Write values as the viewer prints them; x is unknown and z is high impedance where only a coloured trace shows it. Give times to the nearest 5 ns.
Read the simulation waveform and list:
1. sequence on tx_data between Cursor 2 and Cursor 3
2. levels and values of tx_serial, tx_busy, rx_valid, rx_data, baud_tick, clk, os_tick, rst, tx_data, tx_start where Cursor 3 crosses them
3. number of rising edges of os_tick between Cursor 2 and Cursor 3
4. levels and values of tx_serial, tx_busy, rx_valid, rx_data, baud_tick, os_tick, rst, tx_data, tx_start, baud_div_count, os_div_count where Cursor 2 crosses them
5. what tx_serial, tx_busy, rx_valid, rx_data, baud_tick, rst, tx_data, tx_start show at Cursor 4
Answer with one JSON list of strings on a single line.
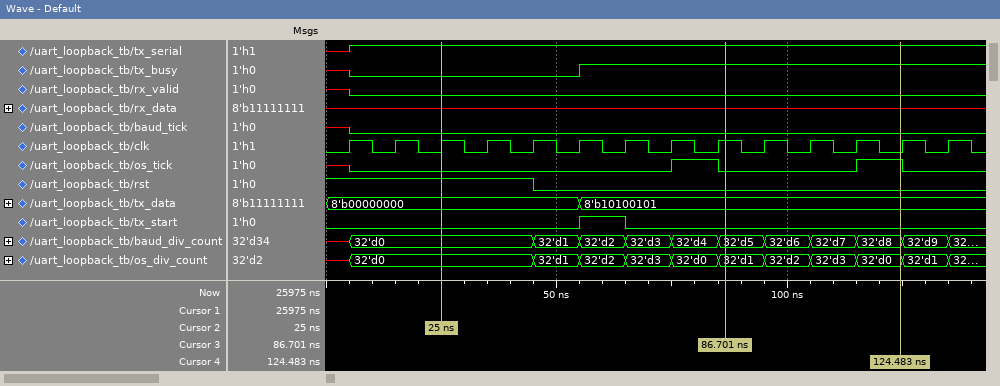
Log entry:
["8'b00000000, 8'b10100101", "tx_serial=1, tx_busy=1, rx_valid=0, rx_data=x, baud_tick=0, clk=1, os_tick=0, rst=0, tx_data=8'b10100101, tx_start=0", "1", "tx_serial=1, tx_busy=0, rx_valid=0, rx_data=x, baud_tick=0, os_tick=0, rst=1, tx_data=8'b00000000, tx_start=0, baud_div_count=32'd0, os_div_count=32'd0", "tx_serial=1, tx_busy=1, rx_valid=0, rx_data=x, baud_tick=0, rst=0, tx_data=8'b10100101, tx_start=0"]
